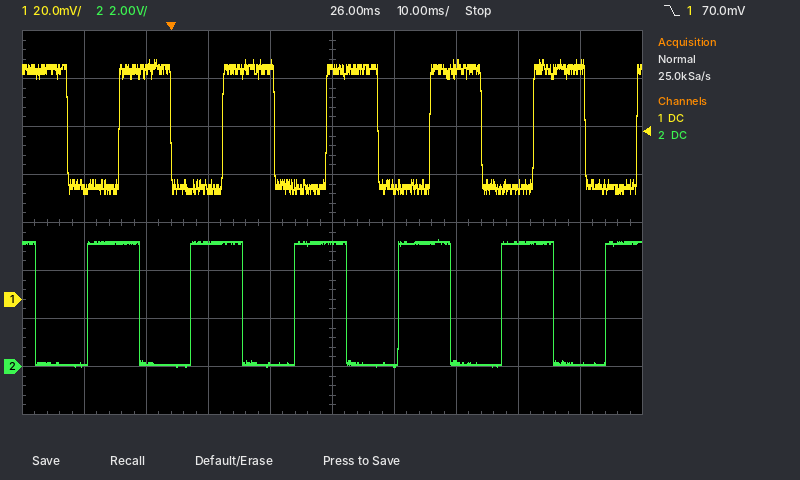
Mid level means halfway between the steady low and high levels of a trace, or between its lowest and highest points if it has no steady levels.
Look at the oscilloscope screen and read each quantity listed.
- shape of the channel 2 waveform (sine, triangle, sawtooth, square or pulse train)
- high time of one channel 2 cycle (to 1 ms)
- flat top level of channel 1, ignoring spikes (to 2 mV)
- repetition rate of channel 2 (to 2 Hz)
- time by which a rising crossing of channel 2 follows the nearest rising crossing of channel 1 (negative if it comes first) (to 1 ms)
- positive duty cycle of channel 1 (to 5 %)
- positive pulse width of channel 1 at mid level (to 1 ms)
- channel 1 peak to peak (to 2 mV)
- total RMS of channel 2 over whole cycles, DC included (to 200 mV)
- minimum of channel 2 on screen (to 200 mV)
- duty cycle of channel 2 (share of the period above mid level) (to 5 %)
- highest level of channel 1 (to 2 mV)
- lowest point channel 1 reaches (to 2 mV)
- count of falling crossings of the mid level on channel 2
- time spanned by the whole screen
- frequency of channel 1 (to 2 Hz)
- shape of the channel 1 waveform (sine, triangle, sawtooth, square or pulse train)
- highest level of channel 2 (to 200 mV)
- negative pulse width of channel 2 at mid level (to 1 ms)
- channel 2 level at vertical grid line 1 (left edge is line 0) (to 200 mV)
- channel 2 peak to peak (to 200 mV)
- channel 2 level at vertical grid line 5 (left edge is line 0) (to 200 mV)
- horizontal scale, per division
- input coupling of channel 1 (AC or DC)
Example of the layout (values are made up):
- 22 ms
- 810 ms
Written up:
- square
- 8 ms
- 96 mV
- 60 Hz
- -5 ms
- 50 %
- 8 ms
- 56 mV
- 3.6 V
- 0.0 V
- 50 %
- 100 mV
- 44 mV
- 6
- 100 ms
- 60 Hz
- square
- 5.2 V
- 8 ms
- 0.0 V
- 5.2 V
- 5.2 V
- 10 ms
- DC
